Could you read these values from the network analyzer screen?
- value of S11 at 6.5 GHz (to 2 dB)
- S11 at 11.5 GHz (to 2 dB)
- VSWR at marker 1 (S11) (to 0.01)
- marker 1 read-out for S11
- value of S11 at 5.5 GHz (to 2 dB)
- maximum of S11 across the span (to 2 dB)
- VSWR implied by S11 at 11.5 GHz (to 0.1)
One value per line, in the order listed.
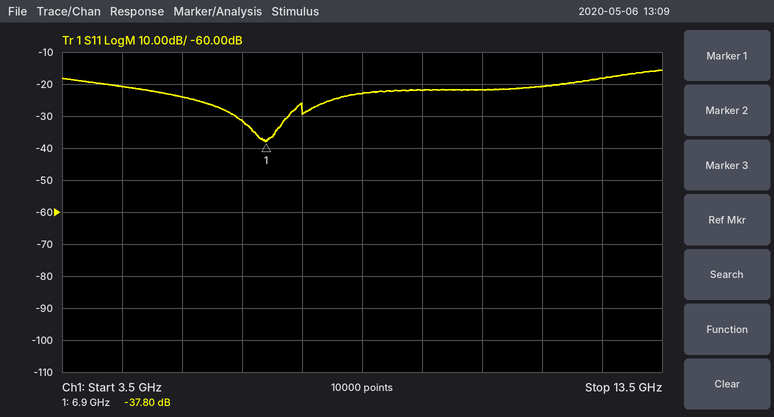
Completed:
-32 dB
-20 dB
1.03
-37.80 dB
-24 dB
-16 dB
1.2
